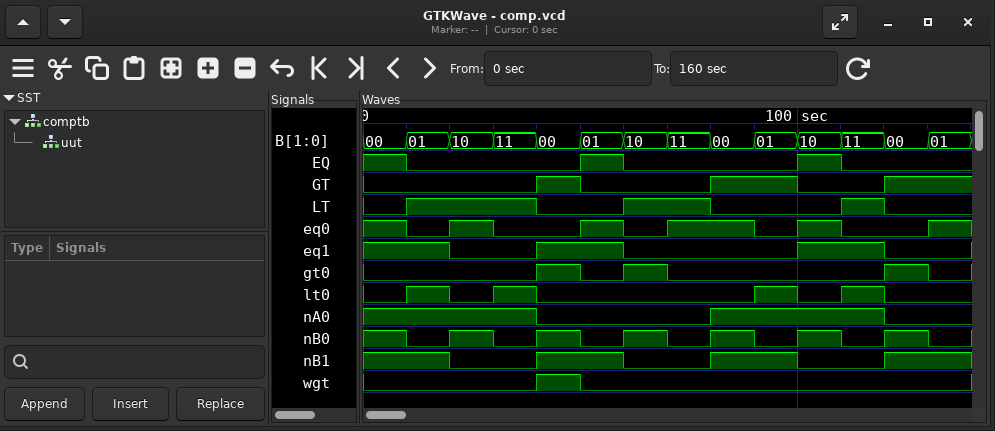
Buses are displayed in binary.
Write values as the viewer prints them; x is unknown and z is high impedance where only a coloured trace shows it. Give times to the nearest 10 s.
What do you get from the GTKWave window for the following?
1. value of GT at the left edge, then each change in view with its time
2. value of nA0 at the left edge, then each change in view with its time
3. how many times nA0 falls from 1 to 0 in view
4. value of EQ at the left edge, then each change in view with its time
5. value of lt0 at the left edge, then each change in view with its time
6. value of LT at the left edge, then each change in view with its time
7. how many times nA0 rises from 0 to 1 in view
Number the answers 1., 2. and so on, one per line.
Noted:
1. 0, 1 at 40 s, 0 at 50 s, 1 at 80 s, 0 at 100 s, 1 at 120 s
2. 1, 0 at 40 s, 1 at 80 s, 0 at 120 s
3. 2
4. 1, 0 at 10 s, 1 at 50 s, 0 at 60 s, 1 at 100 s, 0 at 110 s
5. 0, 1 at 10 s, 0 at 20 s, 1 at 30 s, 0 at 40 s, 1 at 90 s, 0 at 100 s, 1 at 110 s, 0 at 120 s
6. 0, 1 at 10 s, 0 at 40 s, 1 at 60 s, 0 at 80 s, 1 at 110 s, 0 at 120 s
7. 1
